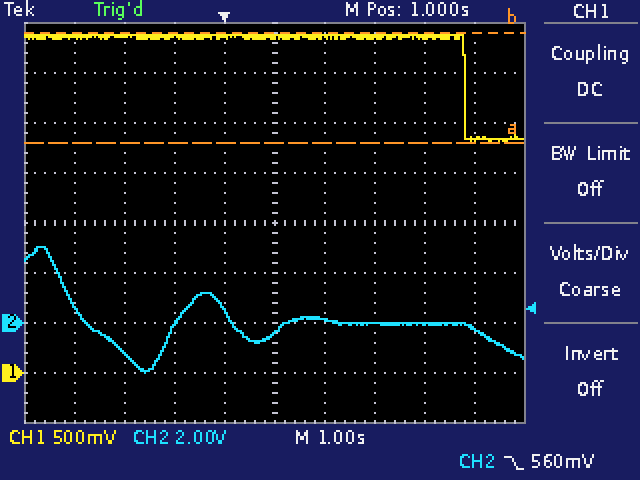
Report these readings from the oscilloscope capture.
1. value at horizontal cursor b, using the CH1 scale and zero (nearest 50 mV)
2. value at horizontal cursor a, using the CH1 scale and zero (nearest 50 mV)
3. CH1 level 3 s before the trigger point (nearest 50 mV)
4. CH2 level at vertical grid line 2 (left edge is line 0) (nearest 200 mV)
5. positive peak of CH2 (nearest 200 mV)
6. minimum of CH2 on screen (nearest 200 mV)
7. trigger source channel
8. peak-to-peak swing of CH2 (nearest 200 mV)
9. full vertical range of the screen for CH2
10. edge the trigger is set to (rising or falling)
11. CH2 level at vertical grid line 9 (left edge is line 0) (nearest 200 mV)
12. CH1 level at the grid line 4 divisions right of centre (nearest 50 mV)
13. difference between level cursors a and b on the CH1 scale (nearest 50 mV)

3.40 V
2.30 V
3.35 V
-1.2 V
3.0 V
-2.0 V
CH2
5.0 V
16 V
falling
-200 mV
2.35 V
1.10 V
